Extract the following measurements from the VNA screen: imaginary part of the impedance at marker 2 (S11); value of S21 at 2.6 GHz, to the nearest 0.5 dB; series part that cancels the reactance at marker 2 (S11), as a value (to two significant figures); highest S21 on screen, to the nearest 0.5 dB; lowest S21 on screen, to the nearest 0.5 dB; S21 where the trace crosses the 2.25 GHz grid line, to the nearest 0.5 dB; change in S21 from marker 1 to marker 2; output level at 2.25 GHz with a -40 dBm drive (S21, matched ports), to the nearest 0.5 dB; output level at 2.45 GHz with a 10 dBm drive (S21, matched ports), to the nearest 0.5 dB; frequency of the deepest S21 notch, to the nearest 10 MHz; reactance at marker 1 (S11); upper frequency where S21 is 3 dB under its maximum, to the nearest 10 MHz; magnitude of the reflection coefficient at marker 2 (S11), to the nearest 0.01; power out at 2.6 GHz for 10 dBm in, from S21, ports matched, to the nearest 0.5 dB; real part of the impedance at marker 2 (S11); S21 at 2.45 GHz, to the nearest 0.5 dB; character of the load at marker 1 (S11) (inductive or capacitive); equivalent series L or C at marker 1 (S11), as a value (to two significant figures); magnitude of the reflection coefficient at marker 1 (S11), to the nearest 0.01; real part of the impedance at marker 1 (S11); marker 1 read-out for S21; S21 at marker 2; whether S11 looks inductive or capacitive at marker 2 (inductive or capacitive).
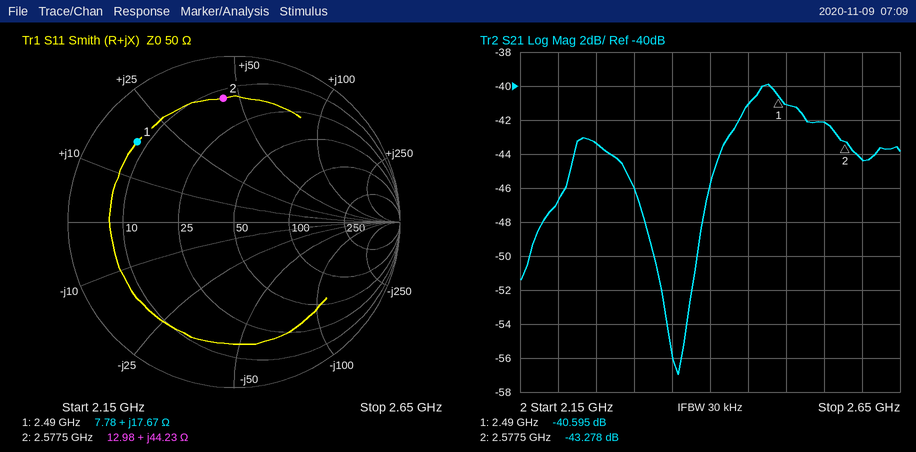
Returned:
+44.23 Ω
-44.5 dB
1.4 pF
-40.0 dB
-57.0 dB
-43.5 dB
-2.683 dB
-83.5 dBm
-31.0 dBm
2.36 GHz
+17.67 Ω
2.57 GHz
0.75
-34.5 dBm
12.98 Ω
-41.0 dB
inductive
1.1 nH
0.76
7.78 Ω
-40.595 dB
-43.278 dB
inductive
